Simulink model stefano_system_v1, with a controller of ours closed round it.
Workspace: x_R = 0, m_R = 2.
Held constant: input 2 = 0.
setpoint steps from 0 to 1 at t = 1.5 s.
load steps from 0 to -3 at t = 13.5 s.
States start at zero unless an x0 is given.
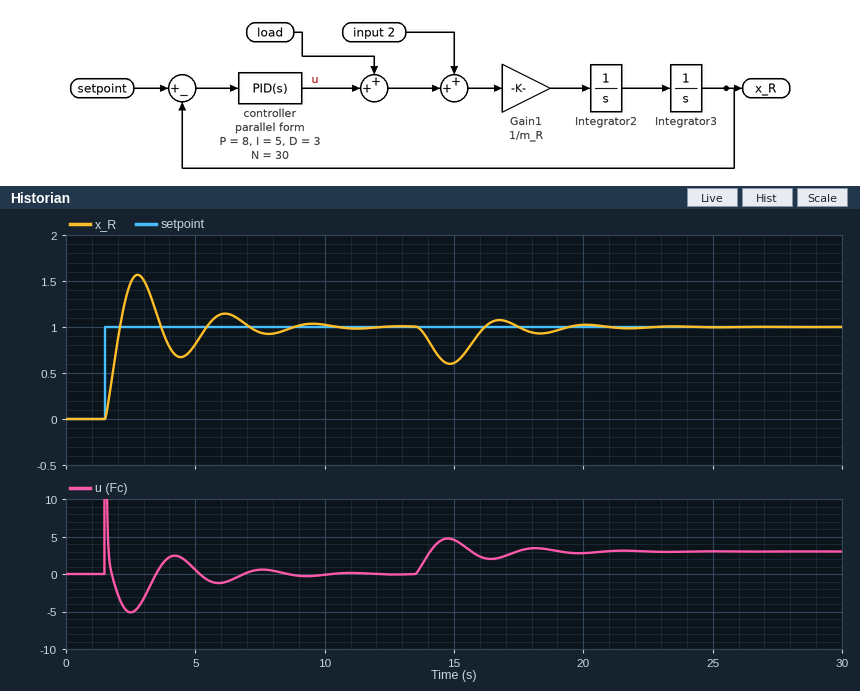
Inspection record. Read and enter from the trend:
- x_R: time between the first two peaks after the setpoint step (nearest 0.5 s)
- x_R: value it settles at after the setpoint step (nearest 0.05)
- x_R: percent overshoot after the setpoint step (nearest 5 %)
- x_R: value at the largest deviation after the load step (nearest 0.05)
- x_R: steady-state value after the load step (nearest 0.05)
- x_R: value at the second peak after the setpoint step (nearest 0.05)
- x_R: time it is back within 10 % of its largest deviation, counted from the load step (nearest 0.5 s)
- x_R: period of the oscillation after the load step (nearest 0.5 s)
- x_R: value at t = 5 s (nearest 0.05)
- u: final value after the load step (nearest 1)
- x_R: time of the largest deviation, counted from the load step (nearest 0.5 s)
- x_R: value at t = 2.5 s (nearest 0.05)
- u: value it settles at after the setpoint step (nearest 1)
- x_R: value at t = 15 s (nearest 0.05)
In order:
3.5 s
1.00
55 %
0.60
1.00
1.15
5.5 s
3.5 s
0.80
3
1.5 s
1.50
0
0.60
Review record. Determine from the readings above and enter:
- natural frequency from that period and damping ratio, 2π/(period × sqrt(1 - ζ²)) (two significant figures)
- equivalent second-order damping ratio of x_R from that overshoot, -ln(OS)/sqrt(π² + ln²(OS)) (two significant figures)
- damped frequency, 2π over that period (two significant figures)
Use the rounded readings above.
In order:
1.8 rad/s
0.19
1.8 rad/s
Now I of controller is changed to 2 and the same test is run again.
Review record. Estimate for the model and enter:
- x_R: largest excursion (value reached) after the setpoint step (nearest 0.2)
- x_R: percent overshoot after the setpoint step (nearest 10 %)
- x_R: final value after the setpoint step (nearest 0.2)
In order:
1.4
50 %
1.0
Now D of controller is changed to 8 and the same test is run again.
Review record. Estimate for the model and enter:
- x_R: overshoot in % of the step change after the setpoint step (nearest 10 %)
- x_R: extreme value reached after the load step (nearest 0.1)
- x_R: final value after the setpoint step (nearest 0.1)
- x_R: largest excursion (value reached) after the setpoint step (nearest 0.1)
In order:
20 %
0.7
1.0
1.2
